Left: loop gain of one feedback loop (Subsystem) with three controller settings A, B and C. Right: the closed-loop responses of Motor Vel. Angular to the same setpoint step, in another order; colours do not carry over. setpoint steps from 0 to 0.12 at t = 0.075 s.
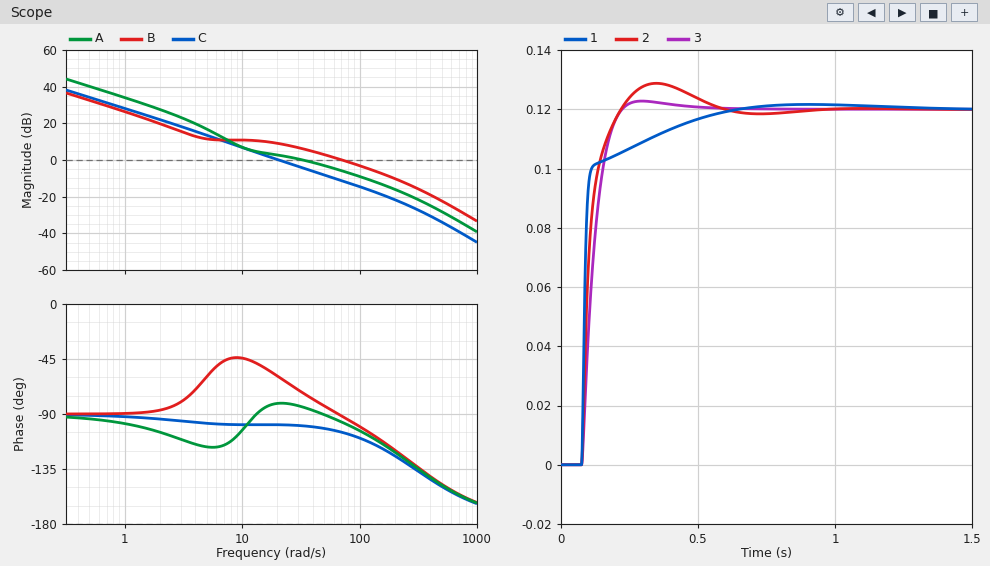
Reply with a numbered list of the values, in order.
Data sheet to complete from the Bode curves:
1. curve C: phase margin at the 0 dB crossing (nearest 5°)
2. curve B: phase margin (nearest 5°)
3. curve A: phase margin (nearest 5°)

1. 80°
2. 90°
3. 95°
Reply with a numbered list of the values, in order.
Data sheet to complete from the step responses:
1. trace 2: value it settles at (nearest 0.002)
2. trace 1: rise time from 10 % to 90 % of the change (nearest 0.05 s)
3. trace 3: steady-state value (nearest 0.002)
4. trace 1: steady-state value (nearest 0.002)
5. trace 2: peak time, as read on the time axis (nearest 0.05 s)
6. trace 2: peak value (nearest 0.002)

1. 0.120
2. 0.20 s
3. 0.120
4. 0.120
5. 0.35 s
6. 0.128
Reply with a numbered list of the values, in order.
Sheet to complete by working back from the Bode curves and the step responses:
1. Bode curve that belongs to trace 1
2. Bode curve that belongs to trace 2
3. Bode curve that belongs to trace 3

1. B
2. A
3. C
